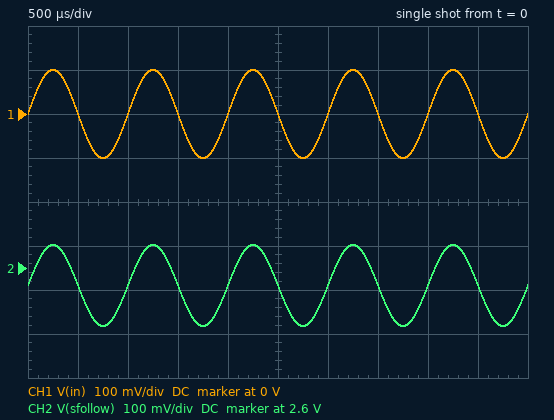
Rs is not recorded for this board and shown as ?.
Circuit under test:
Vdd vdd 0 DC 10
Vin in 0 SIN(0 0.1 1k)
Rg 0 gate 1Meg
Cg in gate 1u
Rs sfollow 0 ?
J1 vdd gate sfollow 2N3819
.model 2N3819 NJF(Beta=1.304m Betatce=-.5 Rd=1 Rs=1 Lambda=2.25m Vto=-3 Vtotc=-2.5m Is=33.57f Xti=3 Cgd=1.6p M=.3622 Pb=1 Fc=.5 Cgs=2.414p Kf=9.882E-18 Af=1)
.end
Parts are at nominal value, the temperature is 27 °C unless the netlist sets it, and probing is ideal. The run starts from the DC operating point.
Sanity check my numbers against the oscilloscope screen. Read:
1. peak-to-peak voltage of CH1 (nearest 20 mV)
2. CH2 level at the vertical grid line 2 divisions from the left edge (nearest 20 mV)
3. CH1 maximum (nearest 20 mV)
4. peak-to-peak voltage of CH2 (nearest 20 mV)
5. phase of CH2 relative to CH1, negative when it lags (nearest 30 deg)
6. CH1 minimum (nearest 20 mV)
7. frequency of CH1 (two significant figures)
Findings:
200 mV
2.56 V
100 mV
180 mV
0 deg
-100 mV
1.0 kHz
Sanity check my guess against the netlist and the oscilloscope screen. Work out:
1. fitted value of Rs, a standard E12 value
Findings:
10 kΩ
